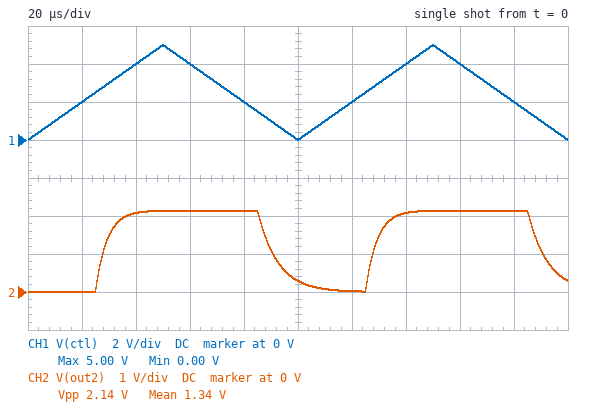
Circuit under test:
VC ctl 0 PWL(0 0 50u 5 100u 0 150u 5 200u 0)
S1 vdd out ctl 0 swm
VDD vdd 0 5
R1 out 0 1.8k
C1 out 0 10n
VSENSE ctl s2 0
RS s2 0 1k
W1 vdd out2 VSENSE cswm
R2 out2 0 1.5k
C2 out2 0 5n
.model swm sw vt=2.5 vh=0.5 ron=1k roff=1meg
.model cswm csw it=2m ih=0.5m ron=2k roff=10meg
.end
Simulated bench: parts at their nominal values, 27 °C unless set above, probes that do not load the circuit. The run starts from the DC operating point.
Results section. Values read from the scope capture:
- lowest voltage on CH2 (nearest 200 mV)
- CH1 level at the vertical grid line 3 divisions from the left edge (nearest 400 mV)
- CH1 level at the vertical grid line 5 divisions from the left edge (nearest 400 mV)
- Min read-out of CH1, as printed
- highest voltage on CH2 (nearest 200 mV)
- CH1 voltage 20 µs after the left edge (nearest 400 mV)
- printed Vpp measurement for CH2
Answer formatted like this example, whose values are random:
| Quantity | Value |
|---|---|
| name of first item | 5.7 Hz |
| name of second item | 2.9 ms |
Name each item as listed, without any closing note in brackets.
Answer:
| Quantity | Value |
|---|---|
| lowest voltage on CH2 | 0 V |
| CH1 level at the vertical grid line 3 divisions from the left edge | 4.0 V |
| CH1 level at the vertical grid line 5 divisions from the left edge | 0 V |
| Min read-out of CH1, as printed | 0.00 V |
| highest voltage on CH2 | 2.2 V |
| CH1 voltage 20 µs after the left edge | 2.0 V |
| printed Vpp measurement for CH2 | 2.14 V |
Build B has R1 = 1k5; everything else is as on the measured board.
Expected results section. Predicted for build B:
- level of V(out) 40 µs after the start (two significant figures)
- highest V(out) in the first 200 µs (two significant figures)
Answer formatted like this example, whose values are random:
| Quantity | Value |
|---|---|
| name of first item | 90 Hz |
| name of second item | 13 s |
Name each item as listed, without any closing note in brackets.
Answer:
| Quantity | Value |
|---|---|
| level of V(out) 40 µs after the start | 2.4 V |
| highest V(out) in the first 200 µs | 3.0 V |
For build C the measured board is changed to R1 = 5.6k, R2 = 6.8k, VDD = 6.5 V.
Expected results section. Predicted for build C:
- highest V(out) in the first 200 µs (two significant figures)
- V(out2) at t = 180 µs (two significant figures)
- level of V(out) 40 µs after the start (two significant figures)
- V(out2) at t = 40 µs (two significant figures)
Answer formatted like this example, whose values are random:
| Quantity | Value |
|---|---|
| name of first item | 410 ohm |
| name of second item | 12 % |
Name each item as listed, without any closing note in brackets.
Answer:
| Quantity | Value |
|---|---|
| highest V(out) in the first 200 µs | 5.5 V |
| V(out2) at t = 180 µs | 5.0 V |
| level of V(out) 40 µs after the start | 3.8 V |
| V(out2) at t = 40 µs | 4.3 V |
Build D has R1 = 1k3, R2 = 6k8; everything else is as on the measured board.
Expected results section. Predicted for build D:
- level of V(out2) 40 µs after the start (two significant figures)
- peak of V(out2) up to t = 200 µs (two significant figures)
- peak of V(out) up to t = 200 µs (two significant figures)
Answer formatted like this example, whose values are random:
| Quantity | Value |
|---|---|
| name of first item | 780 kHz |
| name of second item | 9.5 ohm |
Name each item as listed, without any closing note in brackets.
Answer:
| Quantity | Value |
|---|---|
| level of V(out2) 40 µs after the start | 3.3 V |
| peak of V(out2) up to t = 200 µs | 3.9 V |
| peak of V(out) up to t = 200 µs | 2.8 V |
